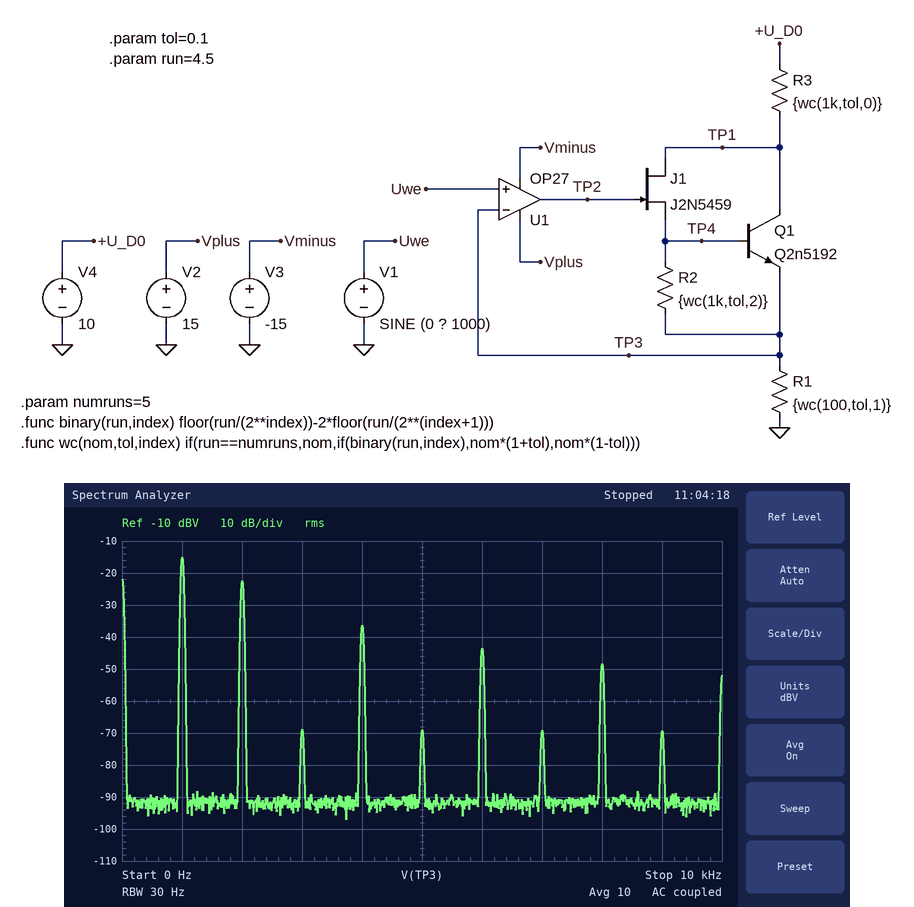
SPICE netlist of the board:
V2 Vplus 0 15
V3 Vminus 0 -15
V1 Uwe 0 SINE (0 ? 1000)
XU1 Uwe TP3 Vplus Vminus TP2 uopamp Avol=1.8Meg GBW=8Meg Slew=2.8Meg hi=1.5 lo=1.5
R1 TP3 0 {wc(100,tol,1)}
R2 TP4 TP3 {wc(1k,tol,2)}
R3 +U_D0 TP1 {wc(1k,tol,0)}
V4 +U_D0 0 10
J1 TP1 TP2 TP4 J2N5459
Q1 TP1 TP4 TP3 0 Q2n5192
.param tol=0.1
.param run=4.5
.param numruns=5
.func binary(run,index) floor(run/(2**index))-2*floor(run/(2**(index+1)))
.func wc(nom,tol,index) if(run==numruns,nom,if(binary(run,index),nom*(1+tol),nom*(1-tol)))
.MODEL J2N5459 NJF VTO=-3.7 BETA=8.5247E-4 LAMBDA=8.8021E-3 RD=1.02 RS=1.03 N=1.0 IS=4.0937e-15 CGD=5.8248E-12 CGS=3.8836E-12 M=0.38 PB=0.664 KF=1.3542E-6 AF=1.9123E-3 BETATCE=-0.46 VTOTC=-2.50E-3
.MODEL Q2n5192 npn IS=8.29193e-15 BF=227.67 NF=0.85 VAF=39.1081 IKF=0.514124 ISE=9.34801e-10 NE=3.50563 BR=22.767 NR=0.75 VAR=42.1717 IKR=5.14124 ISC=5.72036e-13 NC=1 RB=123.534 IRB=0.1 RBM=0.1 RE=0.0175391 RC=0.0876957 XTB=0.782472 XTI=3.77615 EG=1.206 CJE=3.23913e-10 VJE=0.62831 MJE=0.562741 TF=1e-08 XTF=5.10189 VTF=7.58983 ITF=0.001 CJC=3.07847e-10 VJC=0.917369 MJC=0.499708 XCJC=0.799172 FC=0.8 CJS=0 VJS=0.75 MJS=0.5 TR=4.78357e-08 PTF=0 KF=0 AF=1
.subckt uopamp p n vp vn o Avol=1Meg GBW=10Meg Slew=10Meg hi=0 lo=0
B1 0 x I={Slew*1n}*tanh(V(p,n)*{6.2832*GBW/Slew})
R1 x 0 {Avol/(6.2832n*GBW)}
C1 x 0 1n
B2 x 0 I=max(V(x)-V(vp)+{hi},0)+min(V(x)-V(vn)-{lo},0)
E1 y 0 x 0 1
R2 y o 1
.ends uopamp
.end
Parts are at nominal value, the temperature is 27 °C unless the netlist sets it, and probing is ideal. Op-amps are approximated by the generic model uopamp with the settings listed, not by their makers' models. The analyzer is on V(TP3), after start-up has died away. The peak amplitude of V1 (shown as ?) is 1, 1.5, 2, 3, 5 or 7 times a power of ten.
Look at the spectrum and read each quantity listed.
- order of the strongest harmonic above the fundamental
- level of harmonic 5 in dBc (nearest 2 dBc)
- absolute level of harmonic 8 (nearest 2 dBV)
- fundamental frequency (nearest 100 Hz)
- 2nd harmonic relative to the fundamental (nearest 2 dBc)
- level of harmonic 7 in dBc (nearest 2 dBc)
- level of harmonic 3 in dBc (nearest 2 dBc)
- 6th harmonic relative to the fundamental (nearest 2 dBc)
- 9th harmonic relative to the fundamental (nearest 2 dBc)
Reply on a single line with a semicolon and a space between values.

2; -54 dBc; -48 dBV; 1.0 kHz; -8 dBc; -54 dBc; -54 dBc; -28 dBc; -54 dBc
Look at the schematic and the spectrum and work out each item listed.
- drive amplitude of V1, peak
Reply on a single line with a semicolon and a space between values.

500 mV
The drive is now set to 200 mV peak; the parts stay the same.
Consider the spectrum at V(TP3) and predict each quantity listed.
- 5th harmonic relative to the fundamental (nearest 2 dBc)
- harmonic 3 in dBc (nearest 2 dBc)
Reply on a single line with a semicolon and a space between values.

-46 dBc; -46 dBc
